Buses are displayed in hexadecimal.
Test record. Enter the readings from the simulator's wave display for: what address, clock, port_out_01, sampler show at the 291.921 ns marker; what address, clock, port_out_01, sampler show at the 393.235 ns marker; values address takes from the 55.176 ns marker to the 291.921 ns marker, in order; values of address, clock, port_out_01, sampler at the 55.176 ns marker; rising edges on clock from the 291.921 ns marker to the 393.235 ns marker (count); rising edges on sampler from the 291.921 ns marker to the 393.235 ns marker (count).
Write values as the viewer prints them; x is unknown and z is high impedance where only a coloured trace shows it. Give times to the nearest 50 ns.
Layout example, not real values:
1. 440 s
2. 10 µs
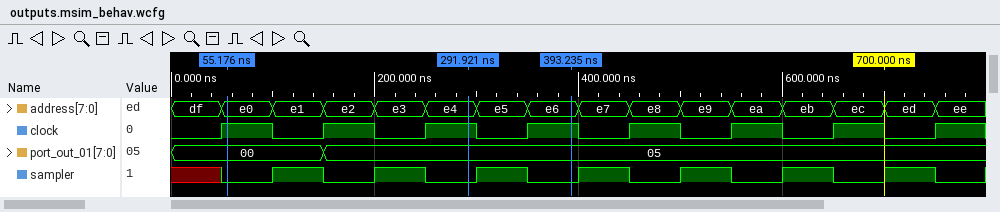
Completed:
1. address=e4, clock=1, port_out_01=05, sampler=0
2. address=e6, clock=1, port_out_01=05, sampler=0
3. e0, e1, e2, e3, e4
4. address=e0, clock=1, port_out_01=00, sampler=0
5. 1
6. 1
